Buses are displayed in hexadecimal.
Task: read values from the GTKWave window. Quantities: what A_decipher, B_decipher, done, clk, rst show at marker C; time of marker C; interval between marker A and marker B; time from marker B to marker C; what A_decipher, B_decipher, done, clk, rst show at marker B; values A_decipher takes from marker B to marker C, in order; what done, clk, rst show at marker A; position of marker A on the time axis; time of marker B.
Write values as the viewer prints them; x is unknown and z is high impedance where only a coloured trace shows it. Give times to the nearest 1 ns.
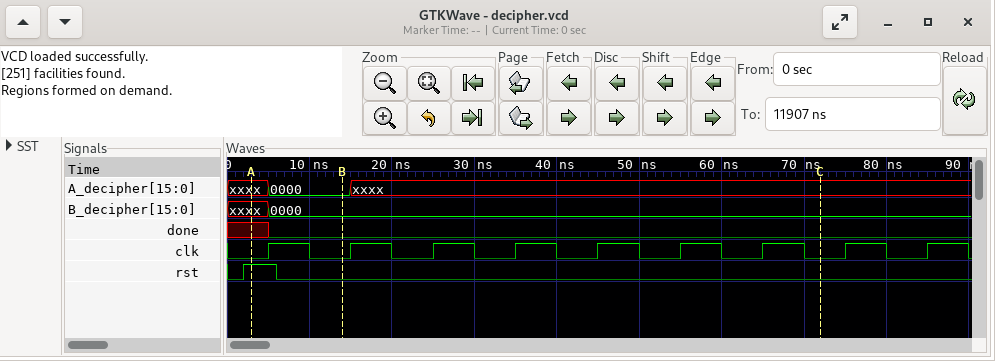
A_decipher=xxxx, B_decipher=0000, done=0, clk=0, rst=0
72 ns
11 ns
58 ns
A_decipher=0000, B_decipher=0000, done=0, clk=0, rst=0
0000, xxxx
done=x, clk=0, rst=1
3 ns
14 ns
